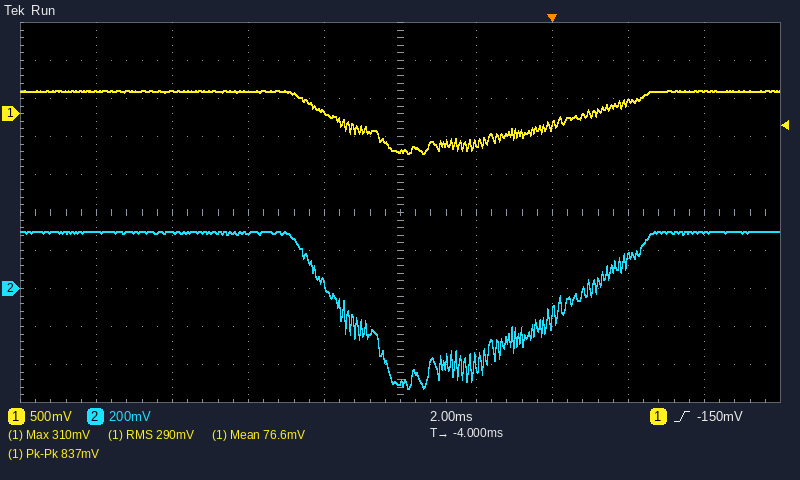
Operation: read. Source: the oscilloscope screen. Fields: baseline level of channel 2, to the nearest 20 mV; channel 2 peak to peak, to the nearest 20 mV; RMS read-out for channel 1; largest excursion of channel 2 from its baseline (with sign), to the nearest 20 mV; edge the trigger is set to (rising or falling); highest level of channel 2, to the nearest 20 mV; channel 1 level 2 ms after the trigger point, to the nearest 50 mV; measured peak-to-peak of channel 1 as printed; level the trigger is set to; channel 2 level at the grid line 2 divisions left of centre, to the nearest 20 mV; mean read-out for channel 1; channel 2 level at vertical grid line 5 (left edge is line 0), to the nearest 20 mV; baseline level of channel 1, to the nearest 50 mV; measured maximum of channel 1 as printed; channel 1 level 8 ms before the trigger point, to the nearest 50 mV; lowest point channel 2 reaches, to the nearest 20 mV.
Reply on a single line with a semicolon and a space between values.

300 mV; 820 mV; 290 mV; -820 mV; rising; 300 mV; 150 mV; 837 mV; -150 mV; 300 mV; 76.6 mV; -500 mV; 300 mV; 310 mV; 300 mV; -520 mV
